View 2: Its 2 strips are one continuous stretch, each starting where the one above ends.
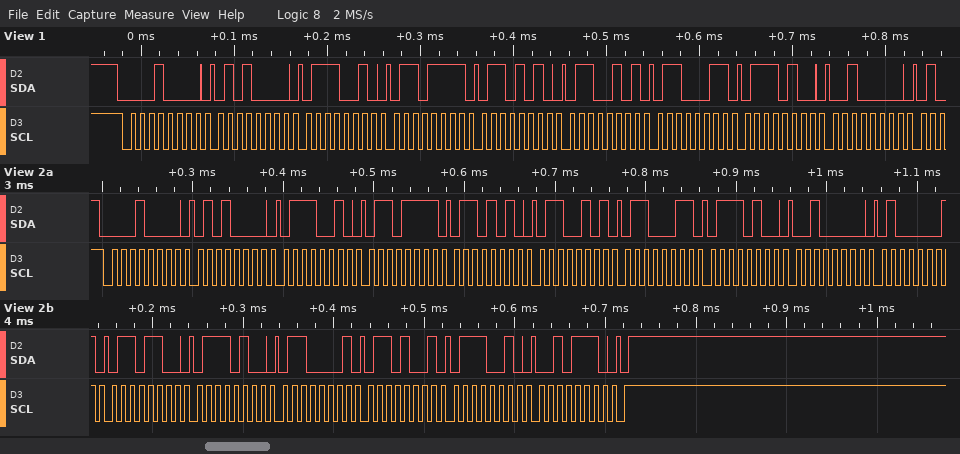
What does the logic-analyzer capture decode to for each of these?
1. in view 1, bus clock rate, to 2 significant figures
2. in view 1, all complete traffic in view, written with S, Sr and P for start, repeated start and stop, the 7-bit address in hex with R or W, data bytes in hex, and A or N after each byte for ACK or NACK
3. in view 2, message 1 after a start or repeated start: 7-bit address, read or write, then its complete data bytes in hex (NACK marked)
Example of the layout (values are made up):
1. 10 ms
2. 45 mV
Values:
1. 100 kHz
2. S 08W A 50 A 72 A 6F A 6A A 65 A 63 A 74 A 20 A
3. 0x08 write: 50 72 6F 6A 65 63 74 20 41 6C 74 61 69 72 2E
